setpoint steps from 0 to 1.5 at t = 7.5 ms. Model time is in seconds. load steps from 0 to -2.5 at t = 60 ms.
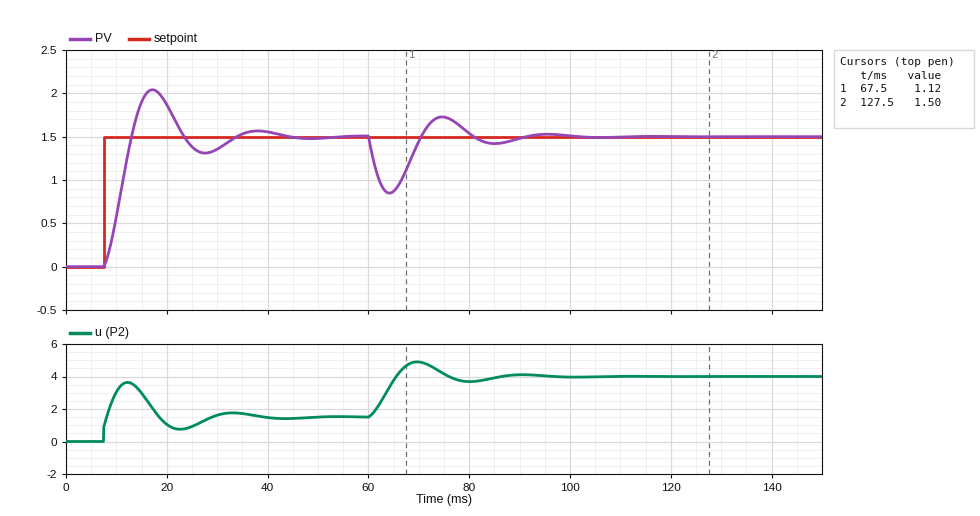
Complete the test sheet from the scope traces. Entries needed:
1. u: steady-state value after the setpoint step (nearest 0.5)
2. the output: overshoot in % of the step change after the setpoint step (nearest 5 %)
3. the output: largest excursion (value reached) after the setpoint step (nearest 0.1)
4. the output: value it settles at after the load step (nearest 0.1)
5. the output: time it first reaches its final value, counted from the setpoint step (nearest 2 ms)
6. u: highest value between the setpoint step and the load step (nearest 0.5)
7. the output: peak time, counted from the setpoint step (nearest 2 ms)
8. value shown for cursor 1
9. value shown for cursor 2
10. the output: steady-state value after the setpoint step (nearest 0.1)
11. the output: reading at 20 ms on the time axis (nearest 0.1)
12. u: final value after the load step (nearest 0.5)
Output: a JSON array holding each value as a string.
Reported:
["1.5", "35 %", "2.0", "1.5", "6 ms", "3.5", "10 ms", "1.12", "1.50", "1.5", "1.9", "4.0"]
